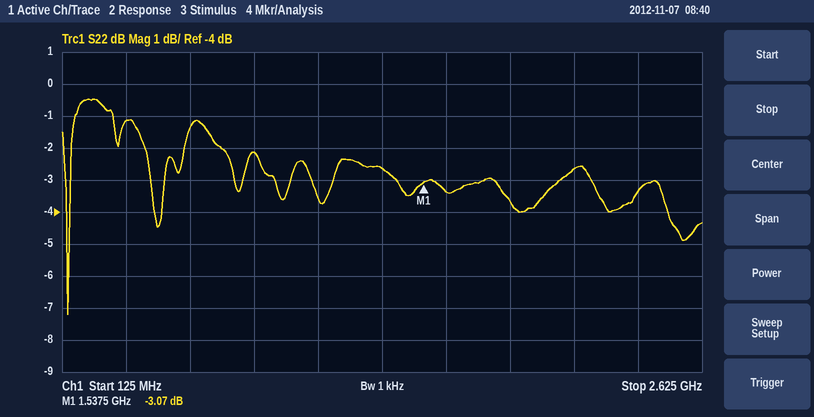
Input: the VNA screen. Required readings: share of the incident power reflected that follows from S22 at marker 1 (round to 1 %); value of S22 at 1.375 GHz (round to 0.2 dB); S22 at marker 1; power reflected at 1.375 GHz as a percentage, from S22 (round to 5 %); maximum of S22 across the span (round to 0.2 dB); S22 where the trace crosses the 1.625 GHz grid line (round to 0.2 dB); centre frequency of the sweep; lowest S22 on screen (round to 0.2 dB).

49 %
-2.6 dB
-3.07 dB
55 %
-0.4 dB
-3.4 dB
1.375 GHz
-7.2 dB
